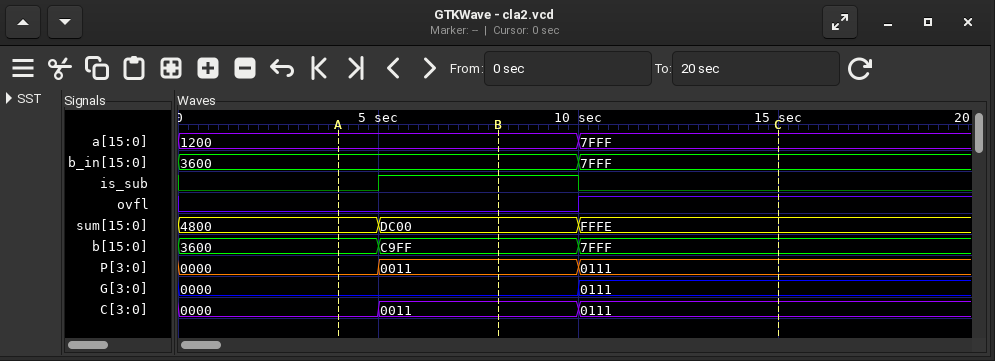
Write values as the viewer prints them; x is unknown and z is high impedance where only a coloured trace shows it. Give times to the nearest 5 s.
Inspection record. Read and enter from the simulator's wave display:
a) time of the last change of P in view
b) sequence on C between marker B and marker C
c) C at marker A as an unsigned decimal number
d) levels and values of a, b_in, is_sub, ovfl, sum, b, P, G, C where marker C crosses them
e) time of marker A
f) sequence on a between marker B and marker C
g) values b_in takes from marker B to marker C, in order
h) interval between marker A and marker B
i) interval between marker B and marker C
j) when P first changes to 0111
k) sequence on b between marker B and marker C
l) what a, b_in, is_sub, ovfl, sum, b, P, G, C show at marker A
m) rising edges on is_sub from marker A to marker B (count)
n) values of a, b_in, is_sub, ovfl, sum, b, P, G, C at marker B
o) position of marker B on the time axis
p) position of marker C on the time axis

10 s
0011, 0111
0
a=7FFF, b_in=7FFF, is_sub=0, ovfl=1, sum=FFFE, b=7FFF, P=0111, G=0111, C=0111
5 s
1200, 7FFF
3600, 7FFF
5 s
5 s
10 s
C9FF, 7FFF
a=1200, b_in=3600, is_sub=0, ovfl=0, sum=4800, b=3600, P=0000, G=0000, C=0000
1
a=1200, b_in=3600, is_sub=1, ovfl=0, sum=DC00, b=C9FF, P=0011, G=0000, C=0011
10 s
15 s
